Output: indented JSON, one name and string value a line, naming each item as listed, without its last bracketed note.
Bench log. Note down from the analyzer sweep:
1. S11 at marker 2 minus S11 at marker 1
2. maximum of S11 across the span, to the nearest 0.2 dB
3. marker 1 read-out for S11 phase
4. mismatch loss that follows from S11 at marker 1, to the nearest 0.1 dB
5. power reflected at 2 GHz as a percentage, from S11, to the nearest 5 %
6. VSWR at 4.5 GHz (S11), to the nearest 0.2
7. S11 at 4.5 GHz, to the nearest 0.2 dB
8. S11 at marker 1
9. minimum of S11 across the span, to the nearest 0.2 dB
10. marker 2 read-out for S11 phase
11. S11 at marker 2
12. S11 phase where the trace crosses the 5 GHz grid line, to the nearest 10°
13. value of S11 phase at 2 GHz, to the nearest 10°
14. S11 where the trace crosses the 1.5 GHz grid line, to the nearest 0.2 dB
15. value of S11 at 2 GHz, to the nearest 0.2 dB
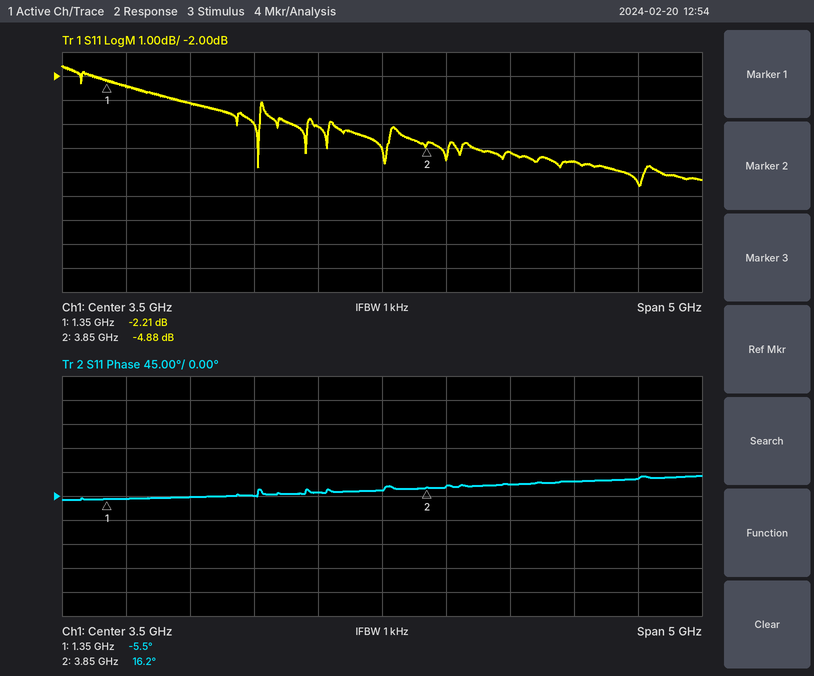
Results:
{
  "S11 at marker 2 minus S11 at marker 1": "-2.67 dB",
  "maximum of S11 across the span, to the nearest 0.2 dB": "-1.6 dB",
  "marker 1 read-out for S11 phase": "-5.5°",
  "mismatch loss that follows from S11 at marker 1, to the nearest 0.1 dB": "4.0 dB",
  "power reflected at 2 GHz as a percentage, from S11, to the nearest 5 %": "50 %",
  "VSWR at 4.5 GHz (S11), to the nearest 0.2": "3.4",
  "S11 at 4.5 GHz, to the nearest 0.2 dB": "-5.2 dB",
  "S11 at marker 1": "-2.21 dB",
  "minimum of S11 across the span, to the nearest 0.2 dB": "-6.6 dB",
  "marker 2 read-out for S11 phase": "16.2°",
  "S11 at marker 2": "-4.88 dB",
  "S11 phase where the trace crosses the 5 GHz grid line, to the nearest 10°": "30°",
  "value of S11 phase at 2 GHz, to the nearest 10°": "0°",
  "S11 where the trace crosses the 1.5 GHz grid line, to the nearest 0.2 dB": "-2.4 dB",
  "value of S11 at 2 GHz, to the nearest 0.2 dB": "-3.2 dB"
}
